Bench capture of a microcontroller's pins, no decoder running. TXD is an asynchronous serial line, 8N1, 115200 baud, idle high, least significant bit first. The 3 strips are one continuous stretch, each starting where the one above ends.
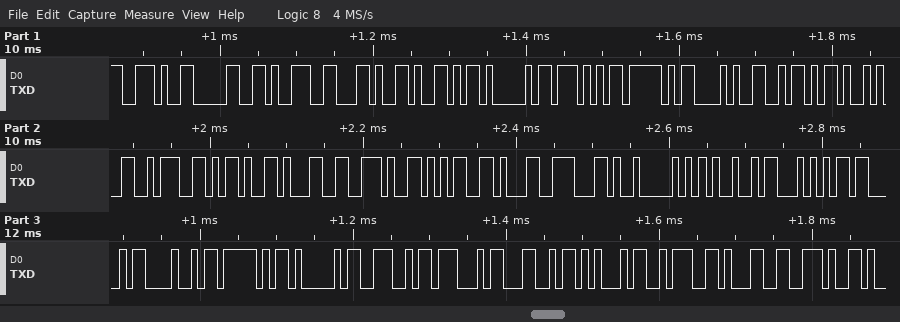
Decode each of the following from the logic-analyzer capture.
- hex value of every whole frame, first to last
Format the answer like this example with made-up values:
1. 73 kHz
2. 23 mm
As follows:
1. 0x2E 0x30 0x39 0x2C 0x59 0x41 0x57 0x5F 0x28 0x5A 0x29 0x3A 0x2D 0x31 0x2E 0x35 0x31 0x2C 0x50 0x49 0x54 0x43 0x48 0x5F 0x41 0x4E 0x47 0x4C 0x45 0x3A 0x31 0x2E
